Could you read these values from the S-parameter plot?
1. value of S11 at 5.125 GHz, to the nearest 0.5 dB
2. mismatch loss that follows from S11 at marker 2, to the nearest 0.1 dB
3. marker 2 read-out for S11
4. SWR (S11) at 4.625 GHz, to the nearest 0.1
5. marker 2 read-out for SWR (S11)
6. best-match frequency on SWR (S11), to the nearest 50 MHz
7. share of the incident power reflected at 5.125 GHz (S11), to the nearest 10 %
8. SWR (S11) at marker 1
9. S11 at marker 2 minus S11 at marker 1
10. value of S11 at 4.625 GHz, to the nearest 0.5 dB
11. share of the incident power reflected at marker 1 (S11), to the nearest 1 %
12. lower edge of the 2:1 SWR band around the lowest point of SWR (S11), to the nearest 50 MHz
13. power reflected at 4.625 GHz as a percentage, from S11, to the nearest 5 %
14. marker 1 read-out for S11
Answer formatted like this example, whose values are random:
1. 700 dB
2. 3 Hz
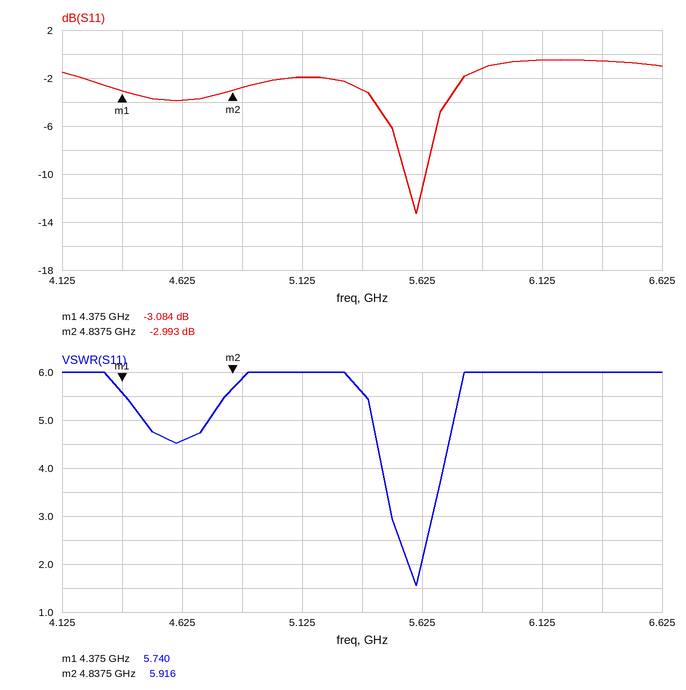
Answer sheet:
1. -2.0 dB
2. 3.0 dB
3. -2.993 dB
4. 4.6
5. 5.916
6. 5.60 GHz
7. 60 %
8. 5.740
9. 0.091 dB
10. -4.0 dB
11. 49 %
12. 5.55 GHz
13. 40 %
14. -3.084 dB
